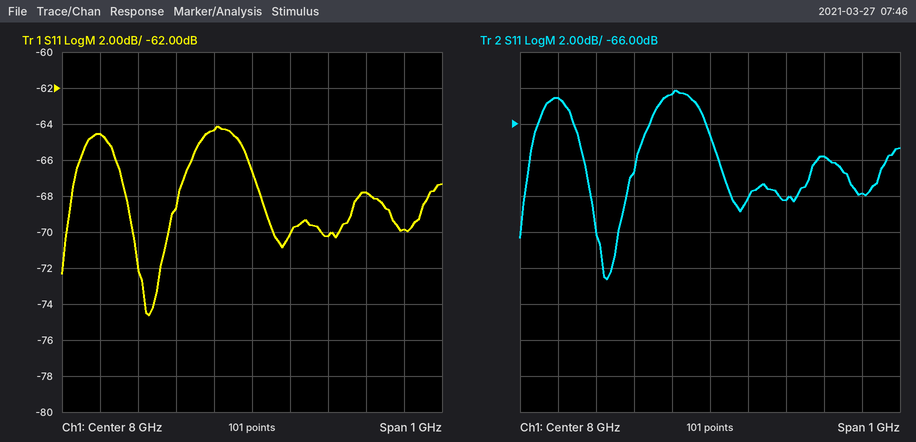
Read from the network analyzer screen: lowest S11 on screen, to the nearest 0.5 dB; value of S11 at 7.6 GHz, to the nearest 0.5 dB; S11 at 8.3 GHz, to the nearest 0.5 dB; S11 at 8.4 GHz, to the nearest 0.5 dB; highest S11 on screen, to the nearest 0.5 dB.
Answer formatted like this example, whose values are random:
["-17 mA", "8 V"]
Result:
["-74.5 dB", "-64.5 dB", "-68.0 dB", "-70.0 dB", "-64.0 dB"]
